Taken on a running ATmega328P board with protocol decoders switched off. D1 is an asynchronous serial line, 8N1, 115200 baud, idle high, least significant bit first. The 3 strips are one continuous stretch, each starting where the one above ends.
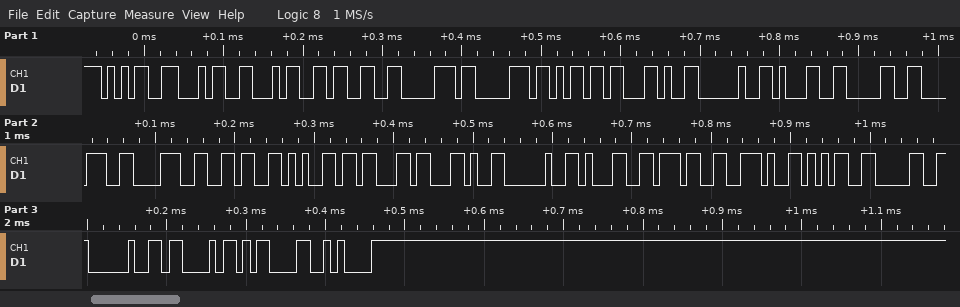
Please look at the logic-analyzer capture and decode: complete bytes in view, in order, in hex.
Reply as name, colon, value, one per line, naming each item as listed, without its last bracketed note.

complete bytes in view, in order, in hex: 35 34 34 33 70 70 6D 2C 20 31 30 38 38 36 65 63 2C 20 31 37 2E 35 30 20 43 0D 0A
